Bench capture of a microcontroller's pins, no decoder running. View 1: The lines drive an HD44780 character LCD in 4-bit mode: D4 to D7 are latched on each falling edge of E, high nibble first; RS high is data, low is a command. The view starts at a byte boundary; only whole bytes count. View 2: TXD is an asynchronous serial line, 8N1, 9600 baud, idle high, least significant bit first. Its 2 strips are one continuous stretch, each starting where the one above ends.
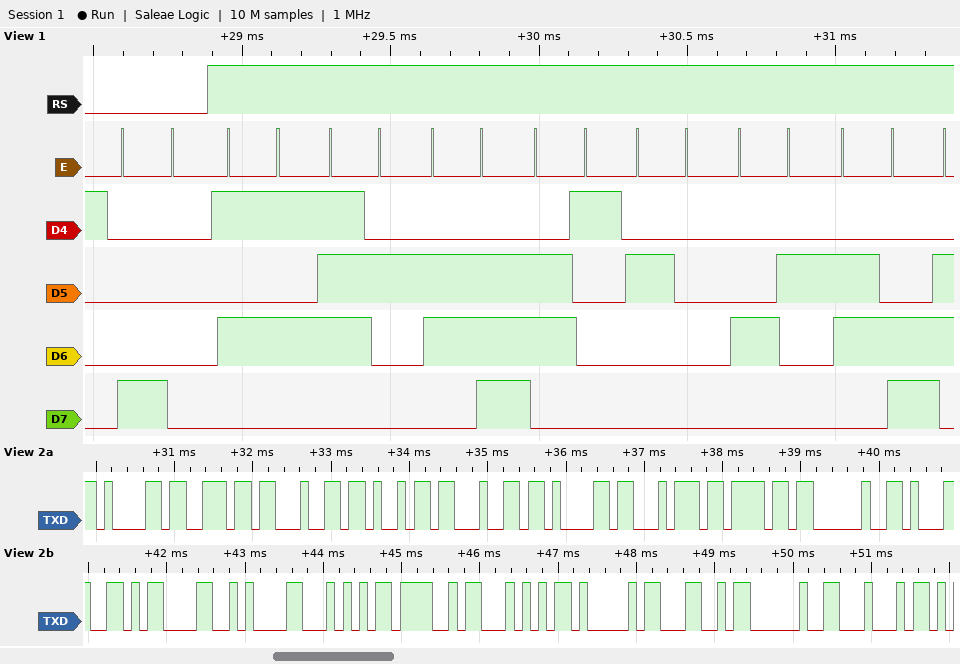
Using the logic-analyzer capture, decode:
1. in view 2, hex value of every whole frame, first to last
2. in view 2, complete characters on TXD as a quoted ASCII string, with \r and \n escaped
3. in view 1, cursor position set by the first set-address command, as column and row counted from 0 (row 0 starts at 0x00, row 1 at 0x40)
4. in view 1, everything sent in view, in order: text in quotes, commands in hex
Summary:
61 6E 64 69 64 61 74 6F 20 31 0D 0A 54 4F 54 41 4C 20 44
"andidato 1\r\nTOTAL D"
column 0, row 0
0x80 "Urna Bl"
